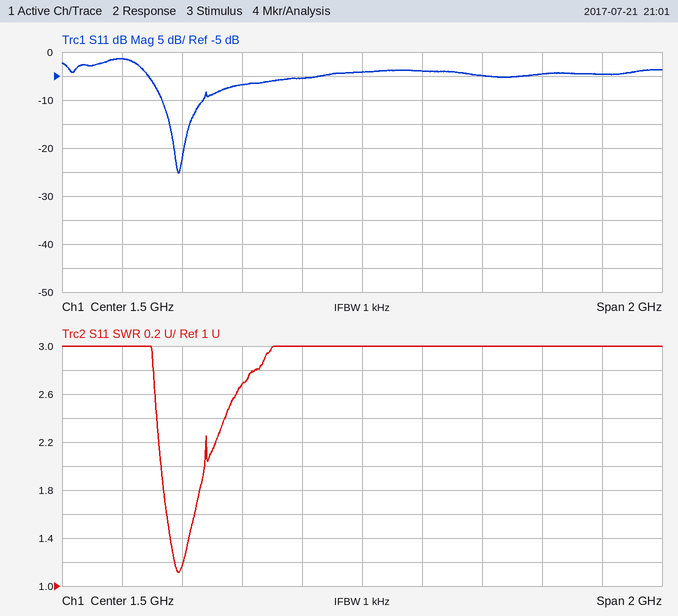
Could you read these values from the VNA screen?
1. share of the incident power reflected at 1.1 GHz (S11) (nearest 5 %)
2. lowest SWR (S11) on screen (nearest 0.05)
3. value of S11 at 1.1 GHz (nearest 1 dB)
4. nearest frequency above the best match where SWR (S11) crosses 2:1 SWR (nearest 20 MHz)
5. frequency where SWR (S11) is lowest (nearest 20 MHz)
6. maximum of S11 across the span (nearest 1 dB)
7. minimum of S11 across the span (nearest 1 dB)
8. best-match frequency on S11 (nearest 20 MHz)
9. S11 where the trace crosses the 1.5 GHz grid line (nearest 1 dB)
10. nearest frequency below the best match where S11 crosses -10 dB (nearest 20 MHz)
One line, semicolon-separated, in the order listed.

20 %; 1.10; -7 dB; 980 MHz; 880 MHz; -1 dB; -25 dB; 880 MHz; -4 dB; 840 MHz
